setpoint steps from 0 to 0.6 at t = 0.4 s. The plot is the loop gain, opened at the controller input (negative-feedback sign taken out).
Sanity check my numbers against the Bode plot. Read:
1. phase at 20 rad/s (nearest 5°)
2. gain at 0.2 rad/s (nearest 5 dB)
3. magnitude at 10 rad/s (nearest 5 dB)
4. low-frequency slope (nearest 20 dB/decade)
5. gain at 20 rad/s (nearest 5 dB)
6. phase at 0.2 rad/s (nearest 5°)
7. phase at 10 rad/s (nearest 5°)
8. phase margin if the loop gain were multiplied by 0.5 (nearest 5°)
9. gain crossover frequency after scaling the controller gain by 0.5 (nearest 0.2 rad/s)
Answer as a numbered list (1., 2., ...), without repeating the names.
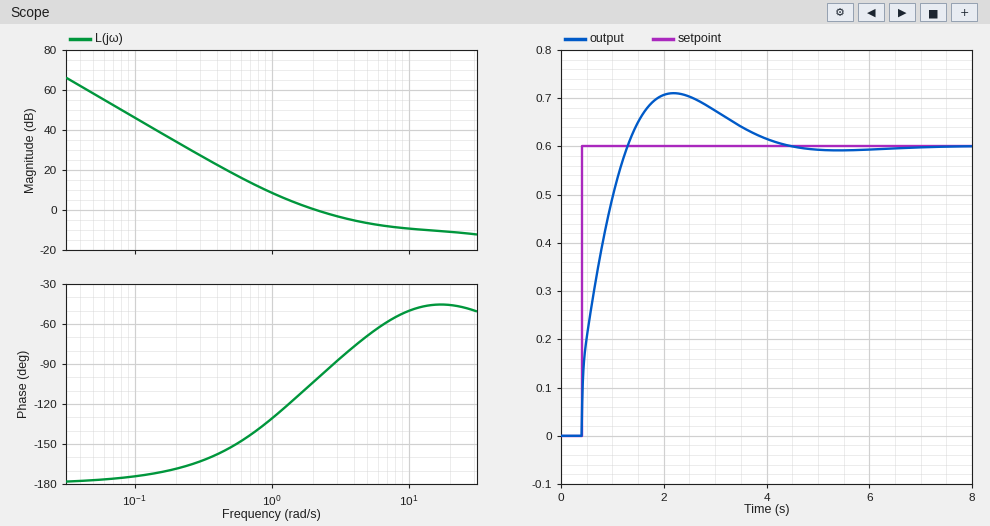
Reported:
1. -45°
2. 35 dB
3. -10 dB
4. -40 dB/decade
5. -10 dB
6. -170°
7. -50°
8. 55°
9. 1.2 rad/s
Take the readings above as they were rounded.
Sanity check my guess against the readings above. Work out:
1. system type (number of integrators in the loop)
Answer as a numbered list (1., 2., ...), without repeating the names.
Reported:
1. 2
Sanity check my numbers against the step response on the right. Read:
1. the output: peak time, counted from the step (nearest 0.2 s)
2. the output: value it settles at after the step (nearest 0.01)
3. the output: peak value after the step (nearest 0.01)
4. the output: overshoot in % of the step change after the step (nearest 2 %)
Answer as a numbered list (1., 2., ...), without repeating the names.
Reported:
1. 1.8 s
2. 0.60
3. 0.71
4. 18 %
